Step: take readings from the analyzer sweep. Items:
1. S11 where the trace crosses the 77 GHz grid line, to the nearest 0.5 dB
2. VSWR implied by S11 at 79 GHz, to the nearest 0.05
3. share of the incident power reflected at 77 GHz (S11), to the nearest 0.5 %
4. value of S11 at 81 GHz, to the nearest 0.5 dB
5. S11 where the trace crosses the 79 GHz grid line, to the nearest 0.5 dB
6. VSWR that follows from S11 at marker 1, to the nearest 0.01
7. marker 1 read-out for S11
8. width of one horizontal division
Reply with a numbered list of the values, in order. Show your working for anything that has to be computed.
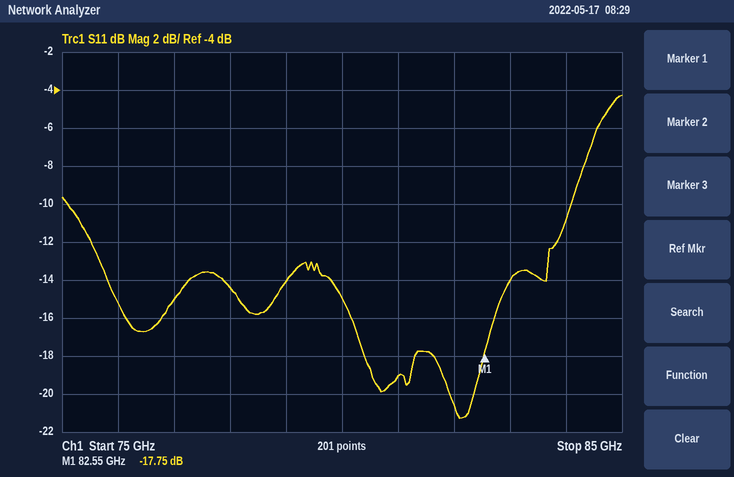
1. -15.0 dB
2. |Γ| = 10^(-14/20) = 0.1995; VSWR = (1 + 0.1995)/(1 − 0.1995) ≈ 1.50
3. 10^(-15/10) ≈ 3.16 %, so 3.0 % to the nearest 0.5 %
4. -19.0 dB
5. -14.0 dB
6. (1 + 0.1296)/(1 − 0.1296) ≈ 1.30
7. -17.75 dB
8. 1 GHz
